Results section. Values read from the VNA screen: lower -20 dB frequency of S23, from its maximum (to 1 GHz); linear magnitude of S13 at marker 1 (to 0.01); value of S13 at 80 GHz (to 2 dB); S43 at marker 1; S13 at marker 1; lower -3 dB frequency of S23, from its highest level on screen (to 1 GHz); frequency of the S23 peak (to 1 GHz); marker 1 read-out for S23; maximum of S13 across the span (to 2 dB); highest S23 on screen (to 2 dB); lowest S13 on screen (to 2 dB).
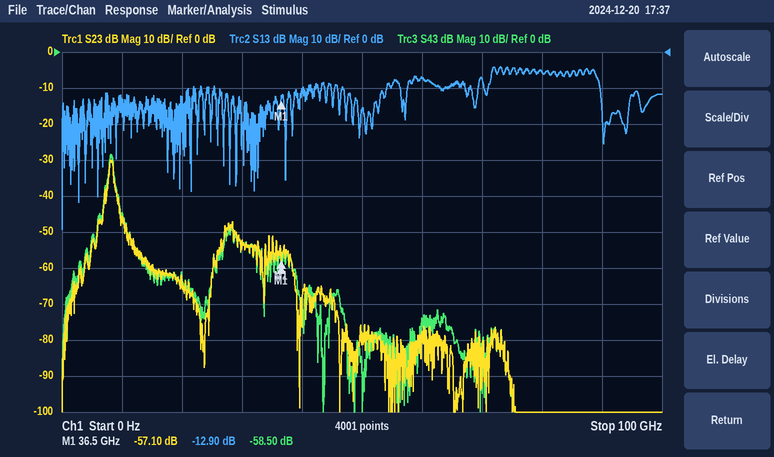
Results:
6 GHz
0.23
-6 dB
-58.50 dB
-12.90 dB
8 GHz
8 GHz
-57.10 dB
-4 dB
-30 dB
-50 dB
